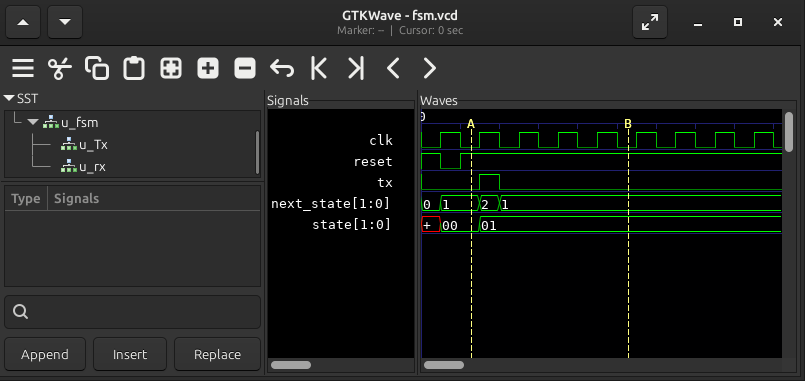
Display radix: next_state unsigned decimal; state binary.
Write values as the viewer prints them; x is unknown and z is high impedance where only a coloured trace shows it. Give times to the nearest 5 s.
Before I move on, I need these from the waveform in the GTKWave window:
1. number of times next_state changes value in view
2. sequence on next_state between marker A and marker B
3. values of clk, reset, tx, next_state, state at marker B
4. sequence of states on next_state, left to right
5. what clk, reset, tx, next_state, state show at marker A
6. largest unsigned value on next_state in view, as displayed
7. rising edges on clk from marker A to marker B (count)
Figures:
3
1, 2, 1
clk=0, reset=1, tx=0, next_state=1, state=01
0, 1, 2, 1
clk=0, reset=1, tx=0, next_state=1, state=00
2
4
